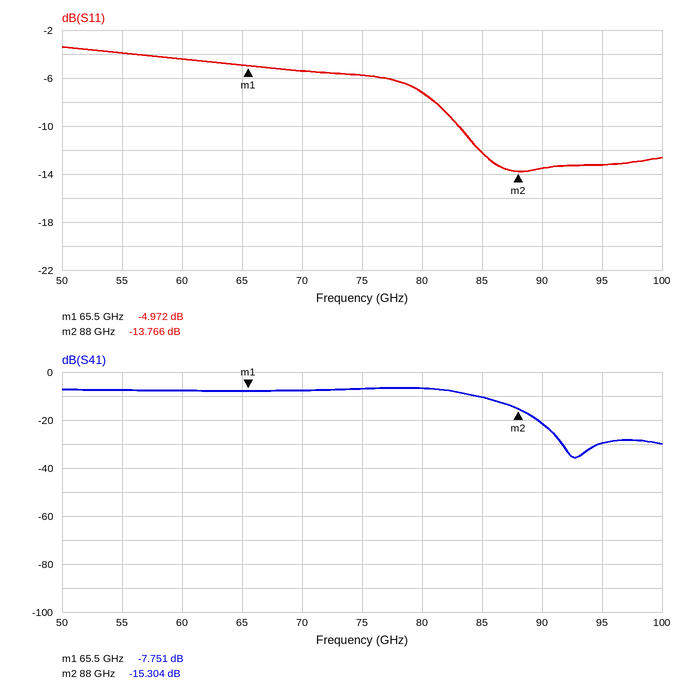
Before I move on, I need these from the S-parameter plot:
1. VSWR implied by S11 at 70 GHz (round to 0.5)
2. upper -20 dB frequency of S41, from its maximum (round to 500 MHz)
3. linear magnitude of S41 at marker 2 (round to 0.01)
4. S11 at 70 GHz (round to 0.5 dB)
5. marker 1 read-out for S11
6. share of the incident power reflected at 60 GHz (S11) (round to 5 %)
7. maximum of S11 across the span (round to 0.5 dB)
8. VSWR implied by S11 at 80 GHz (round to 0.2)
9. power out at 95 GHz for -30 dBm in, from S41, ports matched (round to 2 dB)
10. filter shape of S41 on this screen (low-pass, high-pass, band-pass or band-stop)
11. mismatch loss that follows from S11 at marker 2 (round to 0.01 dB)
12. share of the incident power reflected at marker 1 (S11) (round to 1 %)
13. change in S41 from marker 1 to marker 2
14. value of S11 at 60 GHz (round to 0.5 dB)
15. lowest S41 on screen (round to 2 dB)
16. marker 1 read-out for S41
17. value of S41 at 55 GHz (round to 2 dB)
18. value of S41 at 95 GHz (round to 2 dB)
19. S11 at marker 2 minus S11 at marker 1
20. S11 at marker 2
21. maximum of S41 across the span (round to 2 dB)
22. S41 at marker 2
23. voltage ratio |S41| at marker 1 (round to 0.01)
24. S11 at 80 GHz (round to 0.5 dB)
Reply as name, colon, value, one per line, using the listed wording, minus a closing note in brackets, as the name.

VSWR implied by S11 at 70 GHz: 3.5
upper -20 dB frequency of S41, from its maximum: 91.0 GHz
linear magnitude of S41 at marker 2: 0.17
S11 at 70 GHz: -5.5 dB
marker 1 read-out for S11: -4.972 dB
share of the incident power reflected at 60 GHz (S11): 35 %
maximum of S11 across the span: -3.5 dB
VSWR implied by S11 at 80 GHz: 2.6
power out at 95 GHz for -30 dBm in, from S41, ports matched: -60 dBm
filter shape of S41 on this screen: low-pass
mismatch loss that follows from S11 at marker 2: 0.19 dB
share of the incident power reflected at marker 1 (S11): 32 %
change in S41 from marker 1 to marker 2: -7.553 dB
value of S11 at 60 GHz: -4.5 dB
lowest S41 on screen: -36 dB
marker 1 read-out for S41: -7.751 dB
value of S41 at 55 GHz: -8 dB
value of S41 at 95 GHz: -30 dB
S11 at marker 2 minus S11 at marker 1: -8.794 dB
S11 at marker 2: -13.766 dB
maximum of S41 across the span: -6 dB
S41 at marker 2: -15.304 dB
voltage ratio |S41| at marker 1: 0.41
S11 at 80 GHz: -7.0 dB
